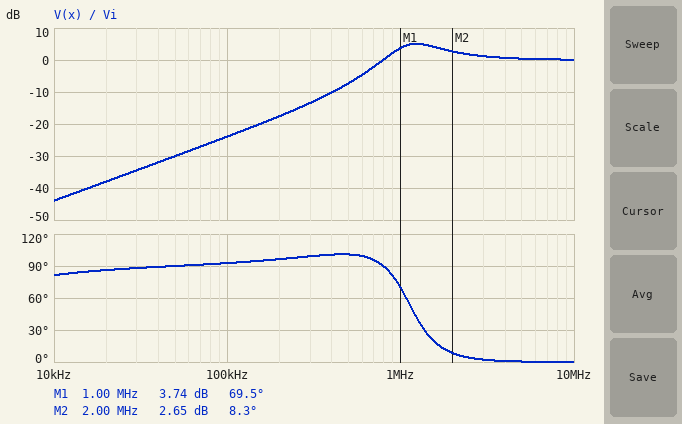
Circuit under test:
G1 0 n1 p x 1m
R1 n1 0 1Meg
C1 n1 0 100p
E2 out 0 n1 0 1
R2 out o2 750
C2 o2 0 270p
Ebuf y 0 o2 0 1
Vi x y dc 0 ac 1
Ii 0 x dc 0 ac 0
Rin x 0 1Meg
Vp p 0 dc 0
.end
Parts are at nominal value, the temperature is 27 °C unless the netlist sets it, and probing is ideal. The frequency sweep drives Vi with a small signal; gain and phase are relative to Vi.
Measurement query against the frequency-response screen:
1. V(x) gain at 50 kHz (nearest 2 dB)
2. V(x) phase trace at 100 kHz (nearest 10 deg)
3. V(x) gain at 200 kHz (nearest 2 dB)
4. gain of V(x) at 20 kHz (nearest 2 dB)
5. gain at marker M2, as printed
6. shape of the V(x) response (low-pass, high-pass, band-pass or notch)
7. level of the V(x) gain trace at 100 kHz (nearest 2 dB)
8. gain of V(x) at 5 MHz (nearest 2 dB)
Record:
-30 dB
90 deg
-18 dB
-38 dB
2.65 dB
high-pass
-24 dB
0 dB
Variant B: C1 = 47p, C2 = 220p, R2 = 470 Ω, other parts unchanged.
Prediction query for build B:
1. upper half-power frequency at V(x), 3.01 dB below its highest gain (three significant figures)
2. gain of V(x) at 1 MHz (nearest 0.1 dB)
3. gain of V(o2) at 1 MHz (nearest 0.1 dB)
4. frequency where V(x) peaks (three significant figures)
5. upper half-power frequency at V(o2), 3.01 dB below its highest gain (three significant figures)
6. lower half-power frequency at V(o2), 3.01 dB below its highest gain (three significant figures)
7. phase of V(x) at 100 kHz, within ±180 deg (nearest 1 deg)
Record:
4.45 MHz
-7.8 dB
1.3 dB
2.49 MHz
2.71 MHz
843 kHz
90 deg
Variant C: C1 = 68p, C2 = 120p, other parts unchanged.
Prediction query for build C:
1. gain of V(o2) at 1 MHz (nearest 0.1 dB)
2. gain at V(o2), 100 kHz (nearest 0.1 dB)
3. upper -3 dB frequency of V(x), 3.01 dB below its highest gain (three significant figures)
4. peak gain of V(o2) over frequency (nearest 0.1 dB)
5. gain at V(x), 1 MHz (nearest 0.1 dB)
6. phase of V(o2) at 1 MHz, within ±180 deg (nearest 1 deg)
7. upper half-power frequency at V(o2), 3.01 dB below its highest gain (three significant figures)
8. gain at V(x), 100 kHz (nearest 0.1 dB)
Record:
1.2 dB
0 dB
6.06 MHz
2.1 dB
-5.0 dB
151 deg
2.41 MHz
-27.4 dB
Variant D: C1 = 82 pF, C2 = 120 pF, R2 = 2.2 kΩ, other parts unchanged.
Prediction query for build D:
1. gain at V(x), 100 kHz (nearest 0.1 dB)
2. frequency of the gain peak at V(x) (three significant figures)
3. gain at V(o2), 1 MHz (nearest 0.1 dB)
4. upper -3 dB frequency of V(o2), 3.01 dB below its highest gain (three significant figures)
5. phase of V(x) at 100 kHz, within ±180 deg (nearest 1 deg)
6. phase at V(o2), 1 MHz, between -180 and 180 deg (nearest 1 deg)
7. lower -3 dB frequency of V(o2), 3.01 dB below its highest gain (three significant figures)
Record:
-25.6 dB
1.15 MHz
5.4 dB
1.27 MHz
95 deg
106 deg
600 kHz
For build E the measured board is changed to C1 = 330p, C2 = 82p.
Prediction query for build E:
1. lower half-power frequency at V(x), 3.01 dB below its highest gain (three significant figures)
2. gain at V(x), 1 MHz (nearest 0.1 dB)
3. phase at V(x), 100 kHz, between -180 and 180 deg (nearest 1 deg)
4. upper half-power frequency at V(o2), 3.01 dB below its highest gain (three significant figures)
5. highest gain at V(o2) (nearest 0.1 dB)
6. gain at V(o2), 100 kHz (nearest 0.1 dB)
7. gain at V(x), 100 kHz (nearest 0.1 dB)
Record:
486 kHz
0.6 dB
80 deg
586 kHz
0 dB
-0.1 dB
-13.8 dB
